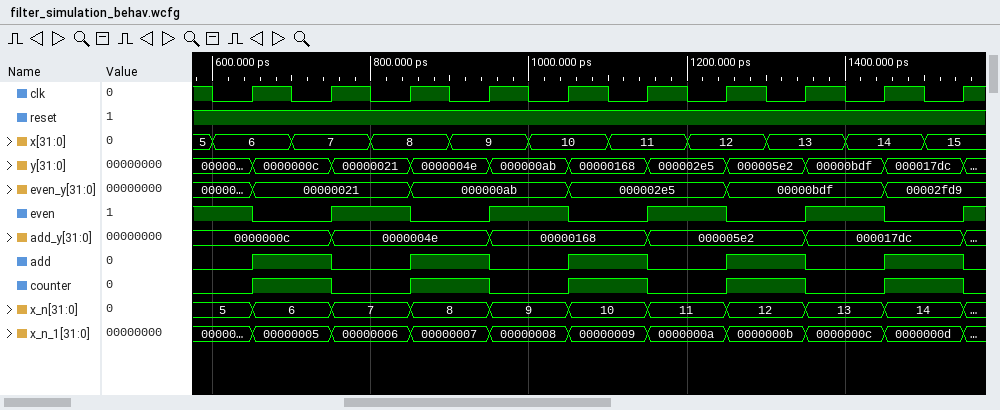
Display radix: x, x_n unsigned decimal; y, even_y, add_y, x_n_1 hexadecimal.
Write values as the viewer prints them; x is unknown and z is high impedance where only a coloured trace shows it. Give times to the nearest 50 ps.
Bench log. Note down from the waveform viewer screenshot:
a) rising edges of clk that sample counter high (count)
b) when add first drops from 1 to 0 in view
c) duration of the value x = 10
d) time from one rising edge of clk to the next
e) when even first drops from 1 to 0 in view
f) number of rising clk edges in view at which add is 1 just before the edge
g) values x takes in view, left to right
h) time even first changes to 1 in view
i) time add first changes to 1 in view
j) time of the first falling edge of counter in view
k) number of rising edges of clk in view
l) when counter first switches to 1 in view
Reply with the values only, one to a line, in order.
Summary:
5
750 ps
100 ps
100 ps
650 ps
5
5, 6, 7, 8, 9, 10, 11, 12, 13, 14, 15
750 ps
650 ps
750 ps
10
650 ps
